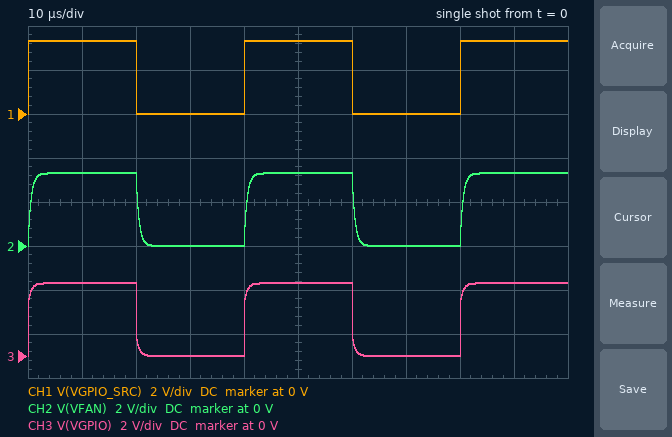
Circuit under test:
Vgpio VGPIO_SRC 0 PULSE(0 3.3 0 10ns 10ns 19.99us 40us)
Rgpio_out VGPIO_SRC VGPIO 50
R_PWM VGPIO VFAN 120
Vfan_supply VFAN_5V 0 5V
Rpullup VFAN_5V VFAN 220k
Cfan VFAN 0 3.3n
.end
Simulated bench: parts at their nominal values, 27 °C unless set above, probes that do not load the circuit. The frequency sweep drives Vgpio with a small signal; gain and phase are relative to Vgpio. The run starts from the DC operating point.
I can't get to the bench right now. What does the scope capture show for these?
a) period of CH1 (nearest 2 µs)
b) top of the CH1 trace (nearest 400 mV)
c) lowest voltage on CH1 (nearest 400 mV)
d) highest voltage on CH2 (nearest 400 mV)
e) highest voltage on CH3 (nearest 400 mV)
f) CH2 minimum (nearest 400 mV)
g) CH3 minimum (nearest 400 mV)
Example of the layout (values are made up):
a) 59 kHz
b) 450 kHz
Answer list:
a) 40 µs
b) 3.2 V
c) 0 V
d) 3.2 V
e) 3.2 V
f) 0 V
g) 0 V
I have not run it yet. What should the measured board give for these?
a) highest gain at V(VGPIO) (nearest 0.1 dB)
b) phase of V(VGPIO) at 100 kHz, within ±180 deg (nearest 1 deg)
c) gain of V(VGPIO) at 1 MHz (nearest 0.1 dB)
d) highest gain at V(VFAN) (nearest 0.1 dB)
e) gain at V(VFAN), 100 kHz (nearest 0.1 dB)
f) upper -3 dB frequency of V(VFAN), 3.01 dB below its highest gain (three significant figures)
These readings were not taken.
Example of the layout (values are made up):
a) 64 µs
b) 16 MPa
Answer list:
a) 0 dB
b) -5 deg
c) -2.7 dB
d) 0 dB
e) -0.5 dB
f) 284 kHz
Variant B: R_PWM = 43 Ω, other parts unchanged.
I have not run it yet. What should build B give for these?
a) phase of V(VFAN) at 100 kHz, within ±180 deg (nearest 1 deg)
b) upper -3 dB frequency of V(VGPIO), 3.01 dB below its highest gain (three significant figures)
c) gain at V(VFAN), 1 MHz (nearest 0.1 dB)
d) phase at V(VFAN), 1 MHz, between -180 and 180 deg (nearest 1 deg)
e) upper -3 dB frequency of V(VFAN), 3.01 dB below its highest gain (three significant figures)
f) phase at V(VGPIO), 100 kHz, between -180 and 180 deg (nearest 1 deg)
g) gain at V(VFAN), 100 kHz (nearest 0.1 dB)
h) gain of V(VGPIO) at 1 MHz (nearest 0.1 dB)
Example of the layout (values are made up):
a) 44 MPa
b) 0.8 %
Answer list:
a) -11 deg
b) 686 kHz
c) -6.7 dB
d) -63 deg
e) 519 kHz
f) -6 deg
g) -0.2 dB
h) -4.2 dB
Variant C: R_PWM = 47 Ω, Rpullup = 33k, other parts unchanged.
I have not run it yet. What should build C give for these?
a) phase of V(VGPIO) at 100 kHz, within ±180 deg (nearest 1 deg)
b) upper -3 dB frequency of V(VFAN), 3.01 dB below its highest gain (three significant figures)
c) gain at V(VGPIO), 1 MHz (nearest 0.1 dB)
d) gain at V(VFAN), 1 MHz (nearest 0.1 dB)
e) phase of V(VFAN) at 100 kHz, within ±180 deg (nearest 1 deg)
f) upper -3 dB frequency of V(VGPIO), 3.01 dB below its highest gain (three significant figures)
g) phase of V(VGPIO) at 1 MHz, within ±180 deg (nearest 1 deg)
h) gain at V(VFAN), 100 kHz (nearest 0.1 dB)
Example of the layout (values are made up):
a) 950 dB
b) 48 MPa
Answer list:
a) -6 deg
b) 499 kHz
c) -4.1 dB
d) -7.0 dB
e) -11 deg
f) 686 kHz
g) -19 deg
h) -0.2 dB
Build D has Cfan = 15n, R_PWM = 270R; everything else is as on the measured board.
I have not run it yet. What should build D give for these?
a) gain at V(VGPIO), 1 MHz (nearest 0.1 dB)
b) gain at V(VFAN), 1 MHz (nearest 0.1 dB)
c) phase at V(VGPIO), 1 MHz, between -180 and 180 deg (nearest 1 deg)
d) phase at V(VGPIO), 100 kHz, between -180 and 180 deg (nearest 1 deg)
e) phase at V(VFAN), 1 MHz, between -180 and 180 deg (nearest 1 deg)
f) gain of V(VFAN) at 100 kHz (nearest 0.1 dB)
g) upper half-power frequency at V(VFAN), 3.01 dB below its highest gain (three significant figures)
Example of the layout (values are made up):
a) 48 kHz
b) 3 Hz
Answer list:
a) -1.5 dB
b) -29.6 dB
c) 0 deg
d) -3 deg
e) -88 deg
f) -10.0 dB
g) 33.2 kHz
